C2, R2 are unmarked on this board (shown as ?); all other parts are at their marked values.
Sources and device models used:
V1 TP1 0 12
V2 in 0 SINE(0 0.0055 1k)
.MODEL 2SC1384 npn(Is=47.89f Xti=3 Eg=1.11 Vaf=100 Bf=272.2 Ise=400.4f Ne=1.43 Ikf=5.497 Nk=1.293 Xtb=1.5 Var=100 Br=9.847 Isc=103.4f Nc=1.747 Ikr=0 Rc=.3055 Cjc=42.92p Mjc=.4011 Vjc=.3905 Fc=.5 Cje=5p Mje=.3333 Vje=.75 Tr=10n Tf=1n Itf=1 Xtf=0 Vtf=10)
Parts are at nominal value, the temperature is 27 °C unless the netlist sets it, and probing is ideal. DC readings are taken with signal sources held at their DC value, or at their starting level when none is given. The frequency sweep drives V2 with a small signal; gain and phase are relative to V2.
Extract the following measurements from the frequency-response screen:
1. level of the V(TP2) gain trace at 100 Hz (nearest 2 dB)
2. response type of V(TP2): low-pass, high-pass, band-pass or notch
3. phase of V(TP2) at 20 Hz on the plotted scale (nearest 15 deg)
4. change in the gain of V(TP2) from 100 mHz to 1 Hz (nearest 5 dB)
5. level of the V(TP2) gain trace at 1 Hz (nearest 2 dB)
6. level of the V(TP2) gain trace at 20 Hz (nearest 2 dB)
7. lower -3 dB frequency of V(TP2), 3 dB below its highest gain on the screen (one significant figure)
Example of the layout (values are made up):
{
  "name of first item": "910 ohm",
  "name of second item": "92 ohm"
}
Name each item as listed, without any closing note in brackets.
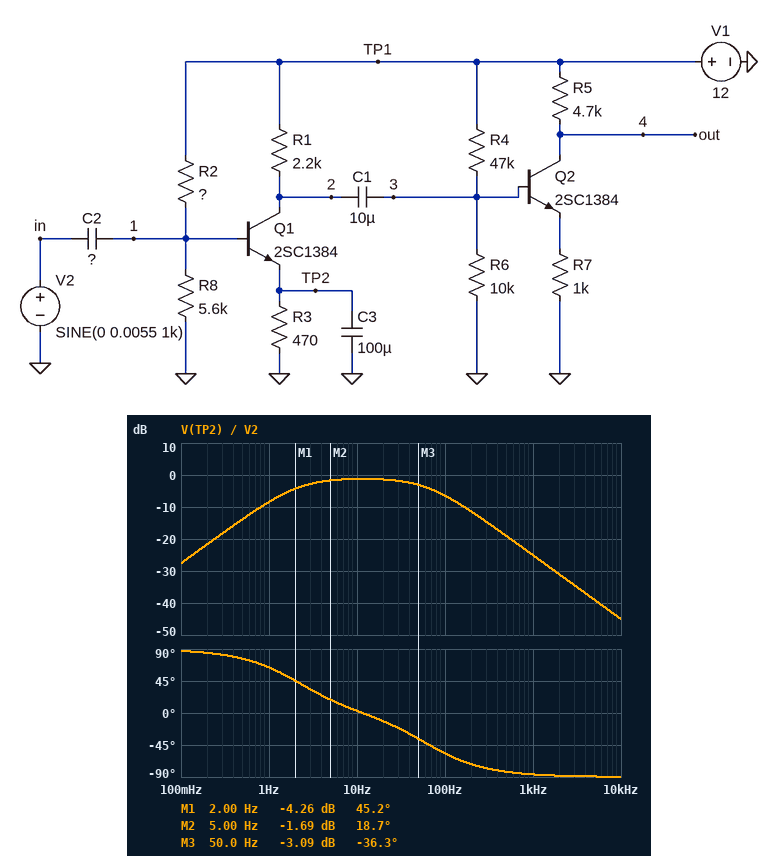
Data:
{
  "level of the V(TP2) gain trace at 100 Hz": "-6 dB",
  "response type of V(TP2): low-pass, high-pass, band-pass or notch": "band-pass",
  "phase of V(TP2) at 20 Hz on the plotted scale": "-15 deg",
  "change in the gain of V(TP2) from 100 mHz to 1 Hz": "20 dB",
  "level of the V(TP2) gain trace at 1 Hz": "-8 dB",
  "level of the V(TP2) gain trace at 20 Hz": "-2 dB",
  "lower -3 dB frequency of V(TP2), 3 dB below its highest gain on the screen": "2 Hz"
}
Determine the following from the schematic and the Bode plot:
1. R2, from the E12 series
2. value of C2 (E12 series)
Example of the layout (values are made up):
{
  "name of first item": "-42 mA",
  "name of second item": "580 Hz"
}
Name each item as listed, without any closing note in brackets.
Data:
{
  "R2, from the E12 series": "56 kΩ",
  "value of C2": "15 µF"
}
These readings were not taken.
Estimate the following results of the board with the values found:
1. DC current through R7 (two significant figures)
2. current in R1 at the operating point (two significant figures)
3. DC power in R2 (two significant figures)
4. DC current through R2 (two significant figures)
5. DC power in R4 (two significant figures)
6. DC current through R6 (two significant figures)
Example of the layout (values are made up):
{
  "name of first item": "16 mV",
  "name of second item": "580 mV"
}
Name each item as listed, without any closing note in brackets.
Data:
{
  "DC current through R7": "1.4 mA",
  "current in R1 at the operating point": "920 µA",
  "DC power in R2": "2.1 mW",
  "DC current through R2": "200 µA",
  "DC power in R4": "2.1 mW",
  "DC current through R6": "200 µA"
}
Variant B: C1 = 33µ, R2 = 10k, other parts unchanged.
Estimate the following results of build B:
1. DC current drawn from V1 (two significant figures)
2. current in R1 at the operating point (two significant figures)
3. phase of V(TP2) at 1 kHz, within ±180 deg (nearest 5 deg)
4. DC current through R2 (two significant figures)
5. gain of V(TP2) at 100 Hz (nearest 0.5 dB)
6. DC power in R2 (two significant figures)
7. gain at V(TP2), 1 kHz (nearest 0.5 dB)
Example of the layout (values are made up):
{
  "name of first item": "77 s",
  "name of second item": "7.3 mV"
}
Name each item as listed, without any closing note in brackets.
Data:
{
  "DC current drawn from V1": "6.9 mA",
  "current in R1 at the operating point": "4.4 mA",
  "phase of V(TP2) at 1 kHz, within ±180 deg": "-70 deg",
  "DC current through R2": "910 µA",
  "gain of V(TP2) at 100 Hz": "-18.0 dB",
  "DC power in R2": "8.2 mW",
  "gain at V(TP2), 1 kHz": "-26.5 dB"
}
